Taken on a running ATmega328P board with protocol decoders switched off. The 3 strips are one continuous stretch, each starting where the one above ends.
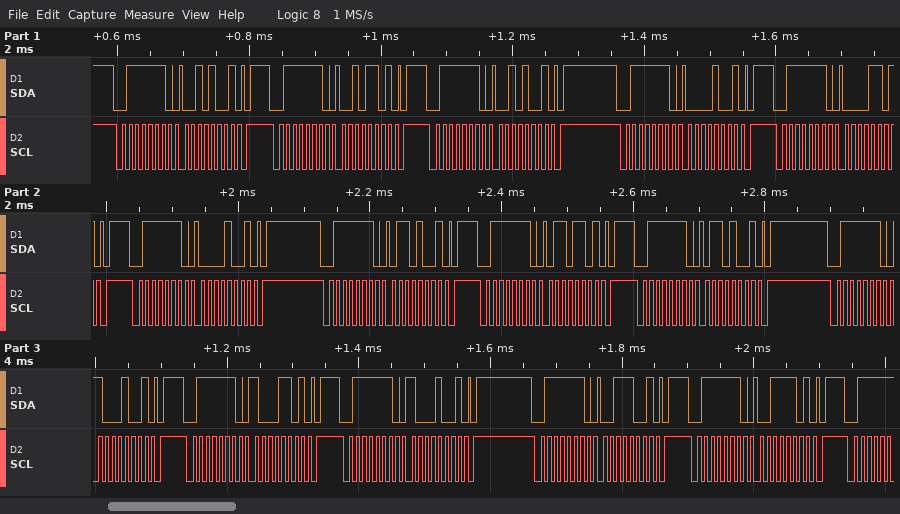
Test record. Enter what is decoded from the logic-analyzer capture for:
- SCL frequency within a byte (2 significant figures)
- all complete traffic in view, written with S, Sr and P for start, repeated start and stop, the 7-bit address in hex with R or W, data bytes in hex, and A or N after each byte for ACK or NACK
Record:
100 kHz
S 3FW A 29 A P S 3FW A 2D A P S 3FW A 29 A P S 3FW A 09 A P S 3FW A 0D A P S 3FW A 09 A P S 3FW A 69 A P S 3FW A 6D A P S 3FW A 69 A P S 3FW A 89 A P S 3FW A 8D A P S 3FW A 89 A P S 3FW A 39 A P S 3FW A 3D A P
